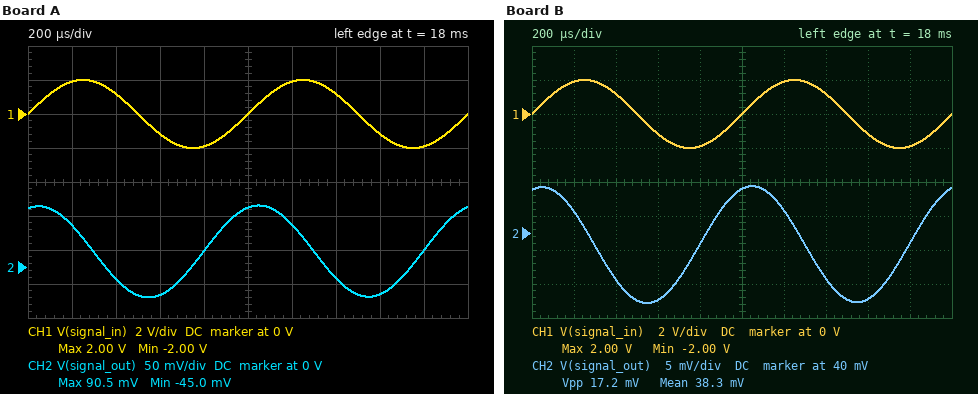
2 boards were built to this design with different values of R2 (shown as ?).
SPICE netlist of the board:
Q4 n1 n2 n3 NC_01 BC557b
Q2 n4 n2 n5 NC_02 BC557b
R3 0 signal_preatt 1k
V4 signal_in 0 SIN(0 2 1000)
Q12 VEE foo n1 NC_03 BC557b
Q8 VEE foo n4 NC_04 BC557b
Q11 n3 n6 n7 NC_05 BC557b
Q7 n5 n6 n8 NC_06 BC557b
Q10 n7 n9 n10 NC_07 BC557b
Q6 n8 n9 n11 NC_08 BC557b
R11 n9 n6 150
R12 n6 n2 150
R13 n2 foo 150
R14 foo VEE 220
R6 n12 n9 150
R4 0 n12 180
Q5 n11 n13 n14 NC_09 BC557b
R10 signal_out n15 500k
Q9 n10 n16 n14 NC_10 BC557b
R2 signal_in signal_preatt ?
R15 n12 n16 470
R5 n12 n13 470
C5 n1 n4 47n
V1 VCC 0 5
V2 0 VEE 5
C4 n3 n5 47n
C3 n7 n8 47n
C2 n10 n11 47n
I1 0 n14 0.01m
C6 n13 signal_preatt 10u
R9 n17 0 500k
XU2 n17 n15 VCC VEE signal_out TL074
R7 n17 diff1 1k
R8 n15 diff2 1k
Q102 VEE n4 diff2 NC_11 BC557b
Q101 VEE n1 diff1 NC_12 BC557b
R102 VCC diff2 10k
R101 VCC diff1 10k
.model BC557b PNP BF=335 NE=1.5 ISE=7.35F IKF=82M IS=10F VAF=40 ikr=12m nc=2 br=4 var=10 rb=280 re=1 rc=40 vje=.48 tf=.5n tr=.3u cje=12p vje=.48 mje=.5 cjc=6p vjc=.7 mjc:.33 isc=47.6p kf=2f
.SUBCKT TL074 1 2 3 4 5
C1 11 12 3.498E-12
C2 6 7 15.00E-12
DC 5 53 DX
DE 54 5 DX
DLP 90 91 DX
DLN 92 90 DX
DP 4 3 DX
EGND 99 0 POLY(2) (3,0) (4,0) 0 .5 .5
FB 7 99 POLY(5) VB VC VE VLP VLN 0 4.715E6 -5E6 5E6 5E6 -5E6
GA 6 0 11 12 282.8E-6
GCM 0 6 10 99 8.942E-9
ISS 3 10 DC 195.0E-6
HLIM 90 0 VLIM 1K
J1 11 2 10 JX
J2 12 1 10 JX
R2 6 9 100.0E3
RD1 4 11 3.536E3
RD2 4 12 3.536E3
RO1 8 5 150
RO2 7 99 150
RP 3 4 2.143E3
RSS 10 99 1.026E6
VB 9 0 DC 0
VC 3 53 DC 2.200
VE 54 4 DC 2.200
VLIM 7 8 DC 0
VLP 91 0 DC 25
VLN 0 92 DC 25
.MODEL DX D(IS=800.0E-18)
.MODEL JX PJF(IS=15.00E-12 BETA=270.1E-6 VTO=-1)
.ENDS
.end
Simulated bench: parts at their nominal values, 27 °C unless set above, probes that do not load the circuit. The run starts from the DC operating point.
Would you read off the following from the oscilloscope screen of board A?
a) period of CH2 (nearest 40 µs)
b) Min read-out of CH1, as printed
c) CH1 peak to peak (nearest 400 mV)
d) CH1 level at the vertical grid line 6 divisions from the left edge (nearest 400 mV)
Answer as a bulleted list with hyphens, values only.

- 1.00 ms
- -2.00 V
- 4.0 V
- 2.0 V
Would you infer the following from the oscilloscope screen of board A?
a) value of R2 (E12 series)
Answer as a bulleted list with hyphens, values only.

- 33 kΩ
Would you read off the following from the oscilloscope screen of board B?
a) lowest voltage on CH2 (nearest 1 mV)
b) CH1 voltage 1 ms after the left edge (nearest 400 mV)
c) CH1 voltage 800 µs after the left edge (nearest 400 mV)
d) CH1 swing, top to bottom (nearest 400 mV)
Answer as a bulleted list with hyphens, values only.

- 30 mV
- 0 V
- -2.0 V
- 4.0 V
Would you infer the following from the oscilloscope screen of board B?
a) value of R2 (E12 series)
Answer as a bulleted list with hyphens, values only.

- 270 kΩ
